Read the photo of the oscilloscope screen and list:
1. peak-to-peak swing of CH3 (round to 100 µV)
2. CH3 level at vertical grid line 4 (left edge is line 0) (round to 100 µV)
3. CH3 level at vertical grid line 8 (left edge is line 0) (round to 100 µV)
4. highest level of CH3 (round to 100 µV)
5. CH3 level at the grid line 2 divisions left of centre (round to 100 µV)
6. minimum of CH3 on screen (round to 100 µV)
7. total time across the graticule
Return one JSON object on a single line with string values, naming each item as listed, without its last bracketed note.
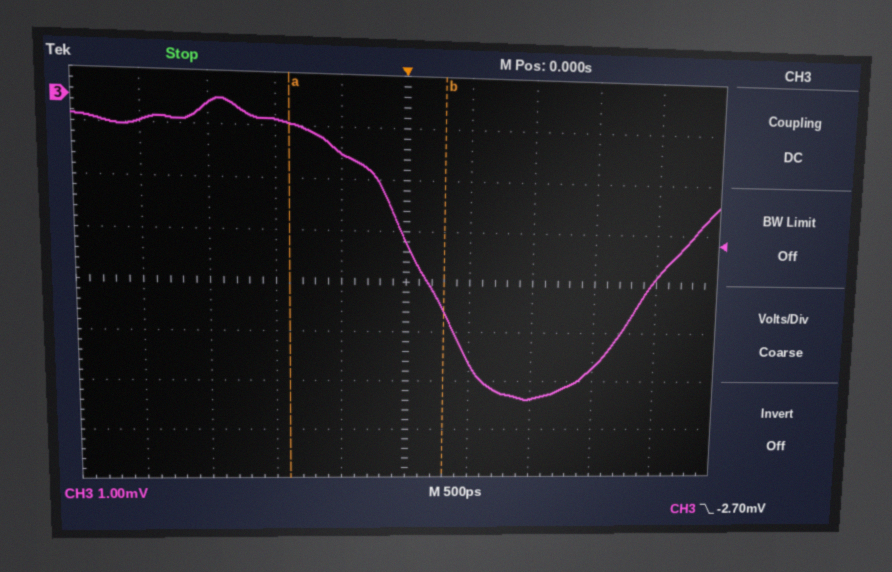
{"peak-to-peak swing of CH3": "5.9 mV", "CH3 level at vertical grid line 4 (left edge is line 0)": "-1.0 mV", "CH3 level at vertical grid line 8 (left edge is line 0)": "-5.2 mV", "highest level of CH3": "0.0 mV", "CH3 level at the grid line 2 divisions left of centre": "-400 µV", "minimum of CH3 on screen": "-5.9 mV", "total time across the graticule": "5 ns"}
